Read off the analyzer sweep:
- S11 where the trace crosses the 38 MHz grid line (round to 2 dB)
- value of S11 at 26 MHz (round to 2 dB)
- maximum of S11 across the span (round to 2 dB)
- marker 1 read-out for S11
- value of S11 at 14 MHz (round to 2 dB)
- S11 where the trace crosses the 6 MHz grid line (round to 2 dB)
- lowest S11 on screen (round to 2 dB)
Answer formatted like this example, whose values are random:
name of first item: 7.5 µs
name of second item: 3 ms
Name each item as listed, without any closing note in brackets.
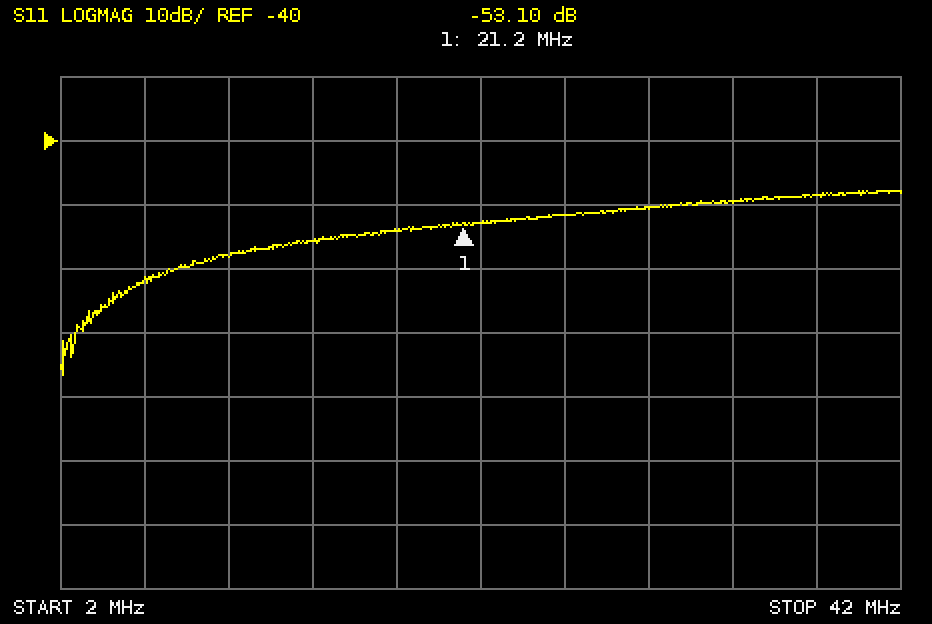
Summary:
S11 where the trace crosses the 38 MHz grid line: -48 dB
value of S11 at 26 MHz: -52 dB
maximum of S11 across the span: -48 dB
marker 1 read-out for S11: -53.10 dB
value of S11 at 14 MHz: -56 dB
S11 where the trace crosses the 6 MHz grid line: -62 dB
lowest S11 on screen: -76 dB
